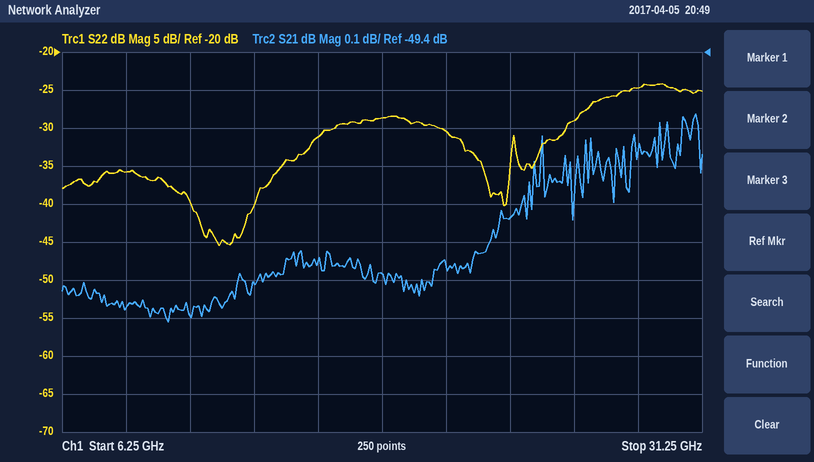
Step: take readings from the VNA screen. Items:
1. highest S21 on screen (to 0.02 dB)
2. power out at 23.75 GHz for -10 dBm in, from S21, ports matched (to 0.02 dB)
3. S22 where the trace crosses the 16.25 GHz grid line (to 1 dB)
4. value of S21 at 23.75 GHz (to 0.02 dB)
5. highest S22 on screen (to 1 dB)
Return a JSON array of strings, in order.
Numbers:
["-49.56 dB", "-59.84 dBm", "-31 dB", "-49.84 dB", "-24 dB"]
